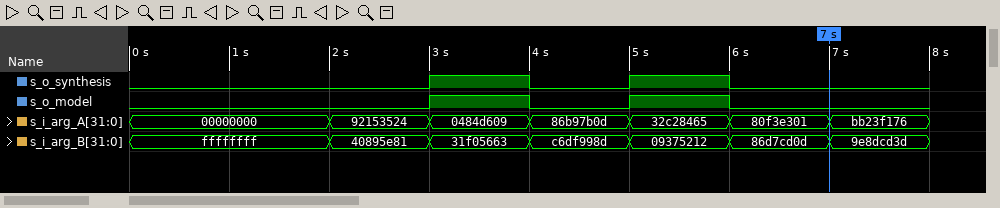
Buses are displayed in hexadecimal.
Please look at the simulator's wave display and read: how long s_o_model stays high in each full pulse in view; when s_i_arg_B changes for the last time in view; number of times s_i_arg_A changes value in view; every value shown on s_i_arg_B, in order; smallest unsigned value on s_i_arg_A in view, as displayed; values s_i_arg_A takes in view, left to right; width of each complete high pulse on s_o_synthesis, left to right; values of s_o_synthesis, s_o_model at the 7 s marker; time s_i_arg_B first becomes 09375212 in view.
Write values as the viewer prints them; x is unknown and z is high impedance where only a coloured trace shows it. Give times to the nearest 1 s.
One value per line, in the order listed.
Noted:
1 s, 1 s
7 s
6
ffffffff, 40895e81, 31f05663, c6df998d, 09375212, 86d7cd0d, 9e8dcd3d
00000000
00000000, 92153524, 0484d609, 86b97b0d, 32c28465, 80f3e301, bb23f176
1 s, 1 s
s_o_synthesis=0, s_o_model=0
5 s
